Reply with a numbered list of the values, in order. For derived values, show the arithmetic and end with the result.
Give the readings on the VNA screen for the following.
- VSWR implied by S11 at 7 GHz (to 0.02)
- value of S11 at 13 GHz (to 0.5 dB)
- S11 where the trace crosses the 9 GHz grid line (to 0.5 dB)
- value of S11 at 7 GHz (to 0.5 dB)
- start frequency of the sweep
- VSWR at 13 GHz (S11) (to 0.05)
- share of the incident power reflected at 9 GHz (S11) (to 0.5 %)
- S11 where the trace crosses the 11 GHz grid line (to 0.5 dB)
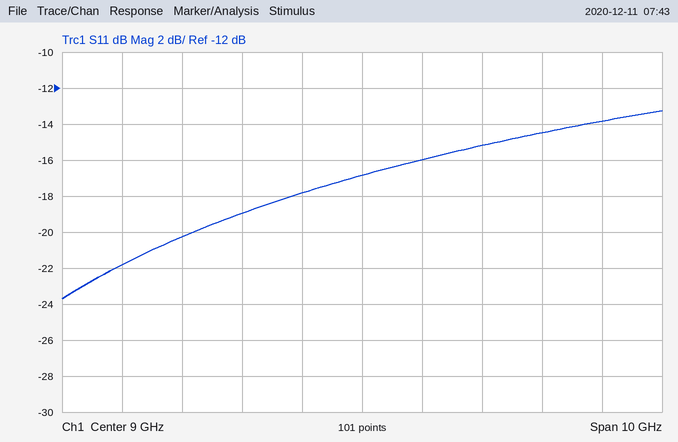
1. |Γ| = 10^(-19/20) = 0.1122; VSWR = (1 + 0.1122)/(1 − 0.1122) ≈ 1.25, so 1.26 to the nearest 0.02
2. -14.0 dB
3. -17.0 dB
4. -19.0 dB
5. 4 GHz
6. |Γ| = 10^(-14/20) = 0.1995; VSWR = (1 + 0.1995)/(1 − 0.1995) ≈ 1.50
7. 10^(-17/10) ≈ 2.0 %
8. -15.0 dB
